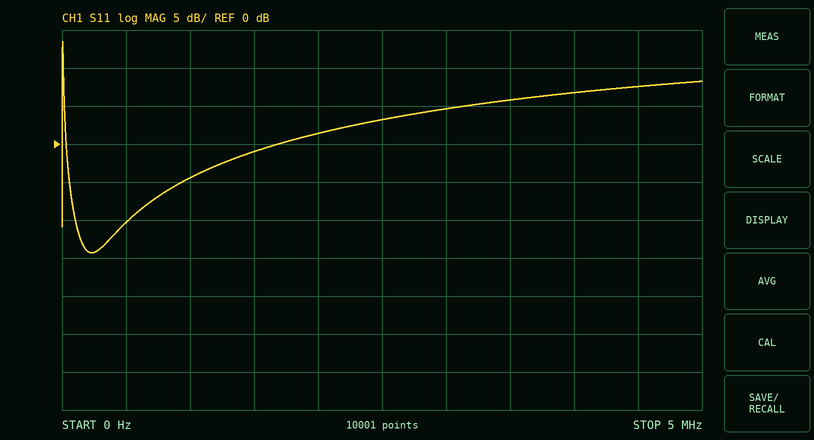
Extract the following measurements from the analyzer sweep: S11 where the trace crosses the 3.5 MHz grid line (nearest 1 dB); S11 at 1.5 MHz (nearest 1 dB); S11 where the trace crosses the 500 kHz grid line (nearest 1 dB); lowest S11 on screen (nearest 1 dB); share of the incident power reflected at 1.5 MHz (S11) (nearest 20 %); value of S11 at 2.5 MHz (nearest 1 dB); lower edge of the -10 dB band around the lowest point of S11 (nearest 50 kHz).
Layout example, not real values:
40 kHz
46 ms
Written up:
6 dB
-1 dB
-10 dB
-14 dB
80 %
3 dB
100 kHz
